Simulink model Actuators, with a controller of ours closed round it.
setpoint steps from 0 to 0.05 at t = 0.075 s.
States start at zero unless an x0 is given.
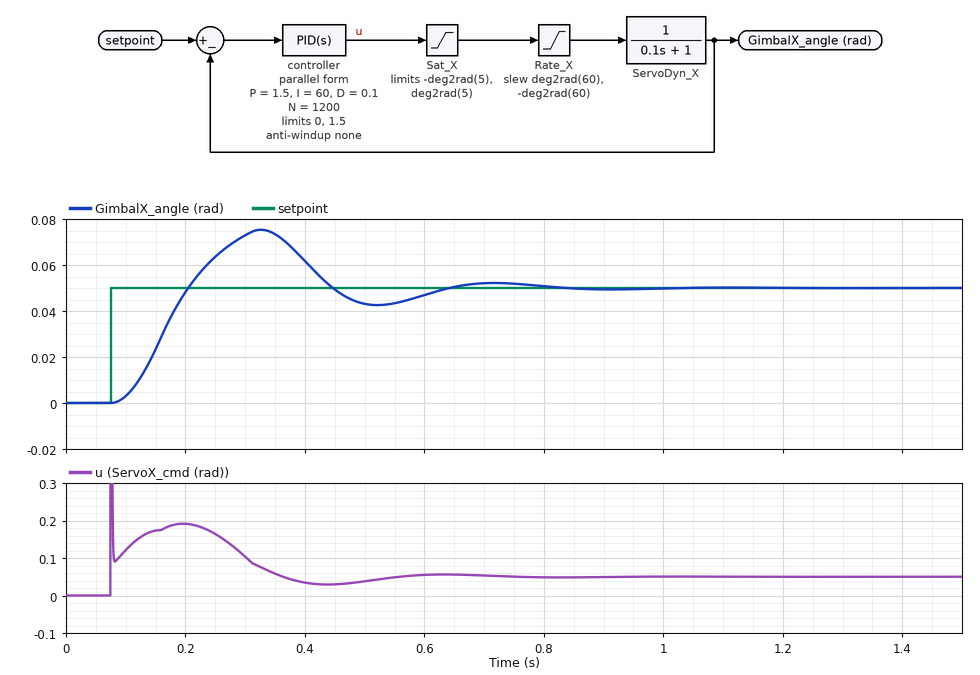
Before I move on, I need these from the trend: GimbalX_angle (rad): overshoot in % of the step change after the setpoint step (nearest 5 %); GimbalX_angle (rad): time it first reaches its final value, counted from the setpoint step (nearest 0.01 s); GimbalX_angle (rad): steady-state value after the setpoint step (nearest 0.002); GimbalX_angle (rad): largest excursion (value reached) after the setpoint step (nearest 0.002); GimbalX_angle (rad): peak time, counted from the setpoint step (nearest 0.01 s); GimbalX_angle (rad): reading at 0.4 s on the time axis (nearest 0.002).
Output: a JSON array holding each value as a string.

["50 %", "0.13 s", "0.050", "0.076", "0.25 s", "0.062"]
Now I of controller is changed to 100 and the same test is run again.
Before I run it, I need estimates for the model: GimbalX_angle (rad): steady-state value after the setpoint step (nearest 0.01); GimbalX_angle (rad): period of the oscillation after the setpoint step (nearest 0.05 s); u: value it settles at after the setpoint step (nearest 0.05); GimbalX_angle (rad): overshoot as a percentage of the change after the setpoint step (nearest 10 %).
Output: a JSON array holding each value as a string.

["0.05", "0.30 s", "0.05", "60 %"]
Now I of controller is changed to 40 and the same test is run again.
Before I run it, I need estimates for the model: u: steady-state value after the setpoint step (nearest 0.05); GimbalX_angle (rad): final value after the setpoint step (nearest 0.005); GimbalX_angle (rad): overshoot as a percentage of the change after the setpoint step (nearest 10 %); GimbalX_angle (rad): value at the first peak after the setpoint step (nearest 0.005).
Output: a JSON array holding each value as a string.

["0.05", "0.050", "40 %", "0.070"]
